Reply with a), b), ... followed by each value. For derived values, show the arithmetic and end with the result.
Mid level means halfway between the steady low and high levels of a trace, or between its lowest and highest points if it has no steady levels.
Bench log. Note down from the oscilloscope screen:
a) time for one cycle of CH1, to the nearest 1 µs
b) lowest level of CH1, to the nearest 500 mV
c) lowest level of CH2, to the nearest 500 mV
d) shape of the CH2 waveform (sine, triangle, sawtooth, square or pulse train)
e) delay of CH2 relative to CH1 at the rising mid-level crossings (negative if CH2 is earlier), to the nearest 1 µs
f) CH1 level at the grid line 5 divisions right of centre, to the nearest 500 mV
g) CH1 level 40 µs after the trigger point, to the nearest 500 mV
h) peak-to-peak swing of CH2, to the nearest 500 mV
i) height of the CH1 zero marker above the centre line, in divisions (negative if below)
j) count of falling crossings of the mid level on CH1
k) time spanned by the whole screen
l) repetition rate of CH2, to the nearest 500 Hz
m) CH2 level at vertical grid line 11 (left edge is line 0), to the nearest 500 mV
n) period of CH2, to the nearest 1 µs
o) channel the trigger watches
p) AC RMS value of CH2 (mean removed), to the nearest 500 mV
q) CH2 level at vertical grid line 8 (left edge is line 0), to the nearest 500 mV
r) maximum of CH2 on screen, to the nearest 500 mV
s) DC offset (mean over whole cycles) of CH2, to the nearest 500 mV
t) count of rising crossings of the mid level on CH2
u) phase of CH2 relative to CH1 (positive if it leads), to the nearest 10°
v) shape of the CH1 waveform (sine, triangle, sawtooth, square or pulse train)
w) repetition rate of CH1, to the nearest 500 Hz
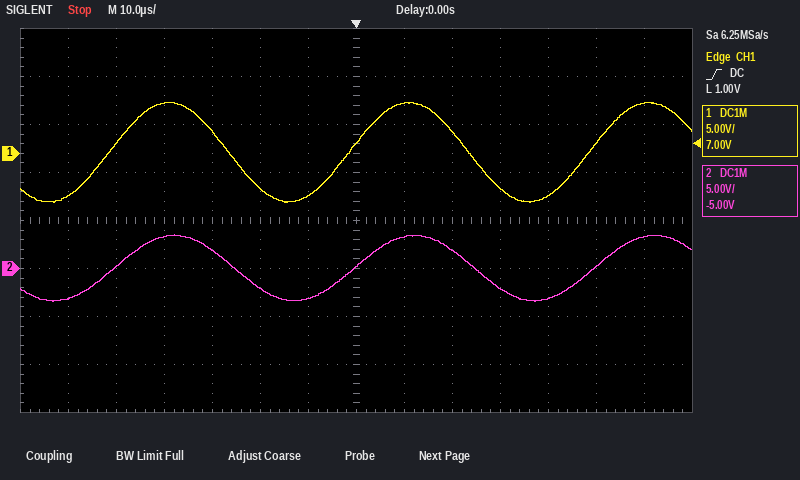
a) 50 µs
b) -5.0 V
c) -3.5 V
d) sine
e) +1 µs
f) 1.0 V
g) -4.5 V
h) 3.5 V − (-3.5 V) = 7.0 V
i) +1.4 div
j) 2
k) 140 µs
l) 1 / 50 µs ≈ 20.0 kHz
m) -3.0 V
n) 50 µs
o) CH1
p) 7.0 V / (2√2) ≈ 2.5 V
q) 3.5 V
r) 3.5 V
s) (3.5 V + (-3.5 V)) / 2 ≈ 0.0 V
t) 3
u) −360° × (+1 µs) / 50 µs ≈ -7.20°, so -10° to the nearest 10°
v) sine
w) 1 / 50 µs ≈ 20.0 kHz
